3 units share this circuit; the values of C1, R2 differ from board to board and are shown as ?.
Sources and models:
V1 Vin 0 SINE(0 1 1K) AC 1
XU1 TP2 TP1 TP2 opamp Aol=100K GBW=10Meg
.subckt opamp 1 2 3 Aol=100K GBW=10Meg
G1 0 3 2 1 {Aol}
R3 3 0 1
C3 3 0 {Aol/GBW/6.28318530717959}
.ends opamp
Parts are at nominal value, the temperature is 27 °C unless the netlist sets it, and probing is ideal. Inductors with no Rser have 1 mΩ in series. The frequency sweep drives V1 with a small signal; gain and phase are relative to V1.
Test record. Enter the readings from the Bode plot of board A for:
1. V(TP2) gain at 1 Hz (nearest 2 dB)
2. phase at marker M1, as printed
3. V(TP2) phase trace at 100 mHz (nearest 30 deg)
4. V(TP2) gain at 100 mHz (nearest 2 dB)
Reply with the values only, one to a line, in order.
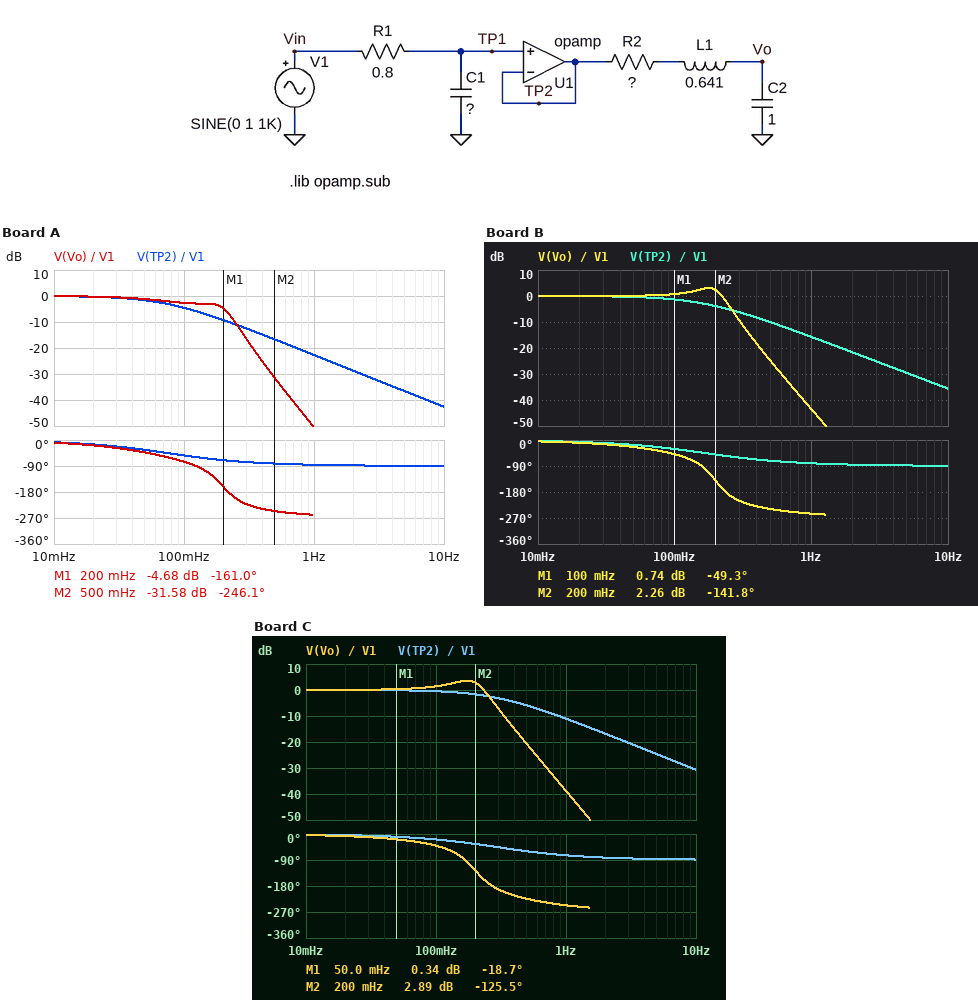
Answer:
-22 dB
-161.0 deg
-60 deg
-4 dB
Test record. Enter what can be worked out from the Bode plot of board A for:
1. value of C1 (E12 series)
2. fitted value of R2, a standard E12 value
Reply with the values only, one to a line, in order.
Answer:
2.7 F
0.47 Ω
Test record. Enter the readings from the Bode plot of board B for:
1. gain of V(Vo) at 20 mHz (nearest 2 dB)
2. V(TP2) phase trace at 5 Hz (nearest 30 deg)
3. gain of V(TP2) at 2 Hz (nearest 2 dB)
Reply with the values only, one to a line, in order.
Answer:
0 dB
-90 deg
-22 dB
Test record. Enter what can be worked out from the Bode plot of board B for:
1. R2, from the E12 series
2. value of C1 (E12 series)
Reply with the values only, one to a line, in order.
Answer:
0.39 Ω
1.2 F
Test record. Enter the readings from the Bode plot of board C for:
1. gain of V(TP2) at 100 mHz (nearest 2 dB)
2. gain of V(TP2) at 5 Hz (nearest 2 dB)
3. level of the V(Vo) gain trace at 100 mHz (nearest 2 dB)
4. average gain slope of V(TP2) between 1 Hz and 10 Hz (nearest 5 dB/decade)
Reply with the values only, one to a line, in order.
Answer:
0 dB
-24 dB
2 dB
-20 dB/decade
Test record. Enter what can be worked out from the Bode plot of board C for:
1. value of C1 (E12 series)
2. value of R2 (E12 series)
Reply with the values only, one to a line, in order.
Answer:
680 mF
0.47 Ω
